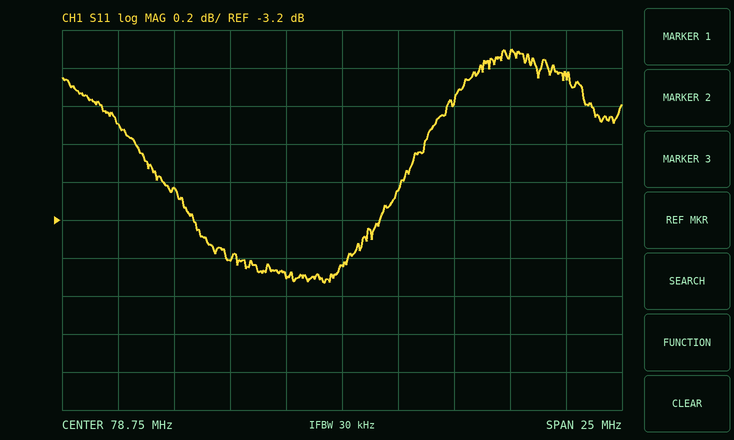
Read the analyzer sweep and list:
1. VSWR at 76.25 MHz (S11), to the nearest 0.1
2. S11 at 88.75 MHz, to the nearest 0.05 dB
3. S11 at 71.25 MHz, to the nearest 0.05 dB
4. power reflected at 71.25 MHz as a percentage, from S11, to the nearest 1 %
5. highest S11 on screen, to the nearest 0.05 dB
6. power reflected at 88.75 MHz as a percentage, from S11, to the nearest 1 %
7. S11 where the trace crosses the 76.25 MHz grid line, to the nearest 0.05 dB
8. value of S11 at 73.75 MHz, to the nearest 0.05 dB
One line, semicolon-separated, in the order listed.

5.0; -2.45 dB; -3.05 dB; 50 %; -2.30 dB; 57 %; -3.50 dB; -3.40 dB
